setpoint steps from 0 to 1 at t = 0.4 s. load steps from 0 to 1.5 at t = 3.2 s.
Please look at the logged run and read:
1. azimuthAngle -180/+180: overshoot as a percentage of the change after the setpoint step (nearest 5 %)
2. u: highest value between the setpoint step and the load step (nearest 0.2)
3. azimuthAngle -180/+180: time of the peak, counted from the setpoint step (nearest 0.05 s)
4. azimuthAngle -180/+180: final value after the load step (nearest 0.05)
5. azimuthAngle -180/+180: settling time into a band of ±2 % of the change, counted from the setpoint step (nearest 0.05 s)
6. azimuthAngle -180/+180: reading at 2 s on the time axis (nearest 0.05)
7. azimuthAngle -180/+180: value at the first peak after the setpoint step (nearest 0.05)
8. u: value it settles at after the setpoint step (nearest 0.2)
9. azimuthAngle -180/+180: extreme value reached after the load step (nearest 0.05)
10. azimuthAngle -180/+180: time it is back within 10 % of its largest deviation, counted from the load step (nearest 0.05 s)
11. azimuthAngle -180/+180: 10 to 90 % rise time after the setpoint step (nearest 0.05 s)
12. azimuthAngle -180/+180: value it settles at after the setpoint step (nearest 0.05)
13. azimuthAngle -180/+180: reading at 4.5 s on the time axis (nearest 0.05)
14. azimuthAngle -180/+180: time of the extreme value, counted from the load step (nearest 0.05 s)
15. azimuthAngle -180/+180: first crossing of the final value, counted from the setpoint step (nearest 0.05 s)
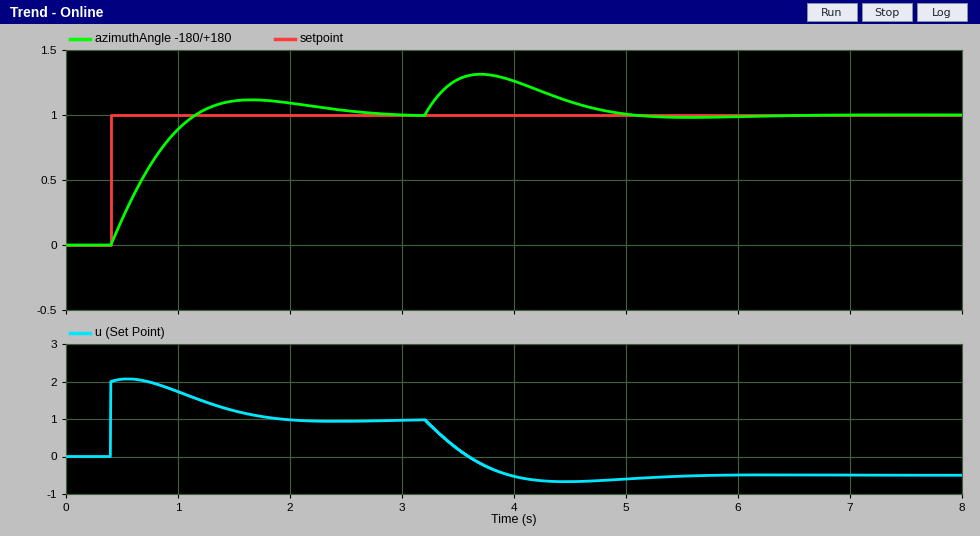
10 %
2.0
1.25 s
1.00
2.25 s
1.10
1.10
1.0
1.30
1.60 s
0.55 s
1.00
1.10
0.50 s
0.75 s
